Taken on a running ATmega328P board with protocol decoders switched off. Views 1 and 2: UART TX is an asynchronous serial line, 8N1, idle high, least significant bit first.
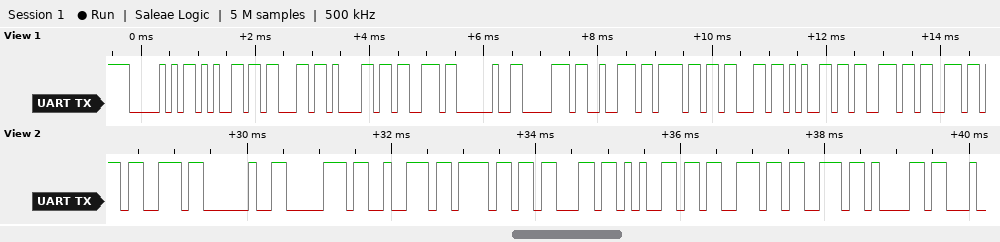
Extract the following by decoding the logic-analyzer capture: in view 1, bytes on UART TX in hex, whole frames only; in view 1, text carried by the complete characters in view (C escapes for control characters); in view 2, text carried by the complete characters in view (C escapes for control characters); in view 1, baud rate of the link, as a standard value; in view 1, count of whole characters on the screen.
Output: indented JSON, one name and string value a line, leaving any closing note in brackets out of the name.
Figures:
{
  "in view 1, bytes on UART TX in hex, whole frames only": "50 65 63 61 73 20 70 72 6F 63 65 73 73",
  "in view 1, text carried by the complete characters in view": "\"Pecas process\"",
  "in view 2, text carried by the complete characters in view": "\"s processa\"",
  "in view 1, baud rate of the link, as a standard value": "9600 baud",
  "in view 1, count of whole characters on the screen": "13"
}
